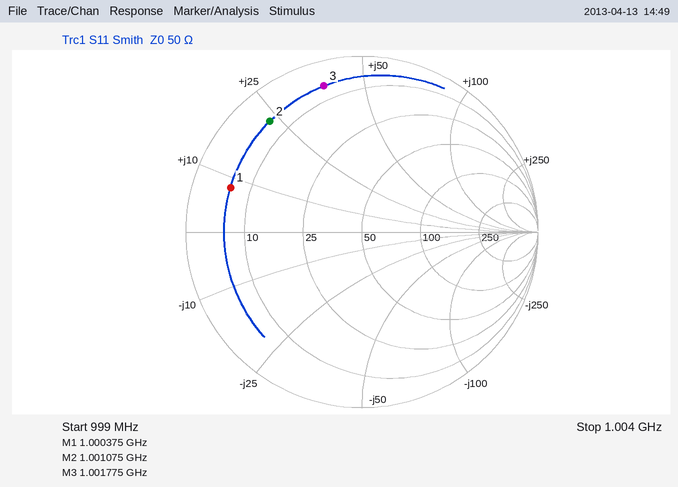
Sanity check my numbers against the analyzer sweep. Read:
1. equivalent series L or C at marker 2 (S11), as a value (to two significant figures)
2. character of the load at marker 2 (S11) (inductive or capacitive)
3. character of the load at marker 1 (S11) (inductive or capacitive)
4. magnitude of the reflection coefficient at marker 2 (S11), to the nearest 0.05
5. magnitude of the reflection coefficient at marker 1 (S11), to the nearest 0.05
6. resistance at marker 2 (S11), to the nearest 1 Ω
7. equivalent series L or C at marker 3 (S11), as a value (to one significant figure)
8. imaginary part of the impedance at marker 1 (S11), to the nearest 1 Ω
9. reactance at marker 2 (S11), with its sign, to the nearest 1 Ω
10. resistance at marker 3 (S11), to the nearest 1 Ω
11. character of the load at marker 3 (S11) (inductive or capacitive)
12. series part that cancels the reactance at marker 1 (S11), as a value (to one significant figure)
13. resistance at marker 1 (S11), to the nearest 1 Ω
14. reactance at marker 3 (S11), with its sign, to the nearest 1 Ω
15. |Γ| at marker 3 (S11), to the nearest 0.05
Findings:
3.7 nH
inductive
inductive
0.80
0.80
6 Ω
6 nH
+8 Ω
+23 Ω
6 Ω
inductive
20 pF
6 Ω
+38 Ω
0.85
